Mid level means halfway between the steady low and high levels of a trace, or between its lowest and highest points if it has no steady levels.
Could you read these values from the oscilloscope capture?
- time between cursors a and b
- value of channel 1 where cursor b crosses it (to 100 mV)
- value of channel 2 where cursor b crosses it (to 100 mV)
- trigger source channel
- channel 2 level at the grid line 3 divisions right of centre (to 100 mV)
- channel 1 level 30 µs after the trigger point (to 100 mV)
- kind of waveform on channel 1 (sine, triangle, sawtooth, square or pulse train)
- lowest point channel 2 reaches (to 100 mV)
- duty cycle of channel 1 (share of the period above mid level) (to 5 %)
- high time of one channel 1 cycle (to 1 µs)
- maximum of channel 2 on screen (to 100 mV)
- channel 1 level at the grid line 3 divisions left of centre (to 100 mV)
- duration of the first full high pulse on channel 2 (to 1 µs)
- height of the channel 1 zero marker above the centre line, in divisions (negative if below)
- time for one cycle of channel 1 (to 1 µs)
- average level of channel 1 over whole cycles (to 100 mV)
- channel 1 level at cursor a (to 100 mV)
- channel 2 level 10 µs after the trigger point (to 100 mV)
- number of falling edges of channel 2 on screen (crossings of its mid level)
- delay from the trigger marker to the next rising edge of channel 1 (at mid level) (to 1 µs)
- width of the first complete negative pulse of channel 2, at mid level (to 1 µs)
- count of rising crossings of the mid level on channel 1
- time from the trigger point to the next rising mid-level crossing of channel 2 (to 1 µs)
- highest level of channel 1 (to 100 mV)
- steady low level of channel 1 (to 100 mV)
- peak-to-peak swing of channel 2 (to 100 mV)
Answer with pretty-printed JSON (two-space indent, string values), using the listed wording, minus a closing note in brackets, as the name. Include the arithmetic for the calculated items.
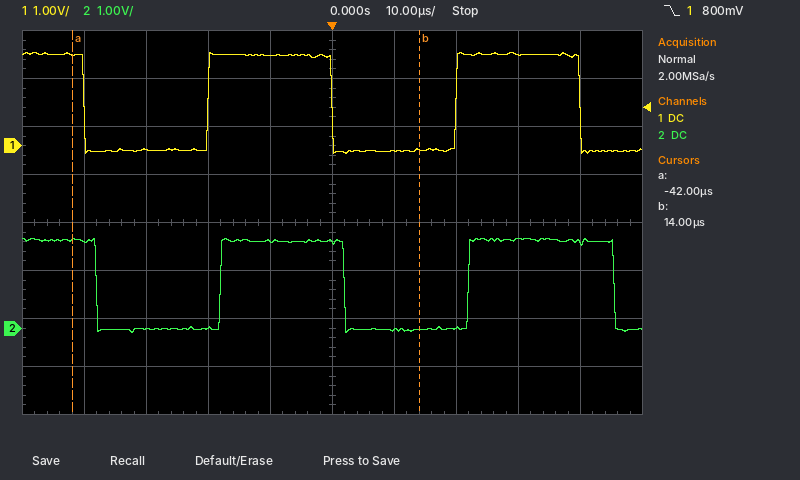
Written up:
{
  "time between cursors a and b": "14 µs − (-42 µs) = 56 µs",
  "value of channel 1 where cursor b crosses it": "-100 mV",
  "value of channel 2 where cursor b crosses it": "0.0 V",
  "trigger source channel": "channel 1",
  "channel 2 level at the grid line 3 divisions right of centre": "1.9 V",
  "channel 1 level 30 µs after the trigger point": "1.9 V",
  "kind of waveform on channel 1": "square",
  "lowest point channel 2 reaches": "-100 mV",
  "duty cycle of channel 1 (share of the period above mid level)": "20 µs / 40 µs ≈ 50 %",
  "high time of one channel 1 cycle": "20 µs",
  "maximum of channel 2 on screen": "1.9 V",
  "channel 1 level at the grid line 3 divisions left of centre": "-100 mV",
  "duration of the first full high pulse on channel 2": "20 µs",
  "height of the channel 1 zero marker above the centre line, in divisions": "+1.6 div",
  "time for one cycle of channel 1": "40 µs",
  "average level of channel 1 over whole cycles": "-100 mV + 0.5 × (1.9 V − (-100 mV)) ≈ 900 mV",
  "channel 1 level at cursor a": "1.9 V",
  "channel 2 level 10 µs after the trigger point": "0.0 V",
  "number of falling edges of channel 2 on screen": "3",
  "delay from the trigger marker to the next rising edge of channel 1 (at mid level)": "20 µs",
  "width of the first complete negative pulse of channel 2, at mid level": "20 µs",
  "count of rising crossings of the mid level on channel 1": "2",
  "time from the trigger point to the next rising mid-level crossing of channel 2": "22 µs",
  "highest level of channel 1": "1.9 V",
  "steady low level of channel 1": "-100 mV",
  "peak-to-peak swing of channel 2": "1.9 V − (-100 mV) = 2.0 V"
}
